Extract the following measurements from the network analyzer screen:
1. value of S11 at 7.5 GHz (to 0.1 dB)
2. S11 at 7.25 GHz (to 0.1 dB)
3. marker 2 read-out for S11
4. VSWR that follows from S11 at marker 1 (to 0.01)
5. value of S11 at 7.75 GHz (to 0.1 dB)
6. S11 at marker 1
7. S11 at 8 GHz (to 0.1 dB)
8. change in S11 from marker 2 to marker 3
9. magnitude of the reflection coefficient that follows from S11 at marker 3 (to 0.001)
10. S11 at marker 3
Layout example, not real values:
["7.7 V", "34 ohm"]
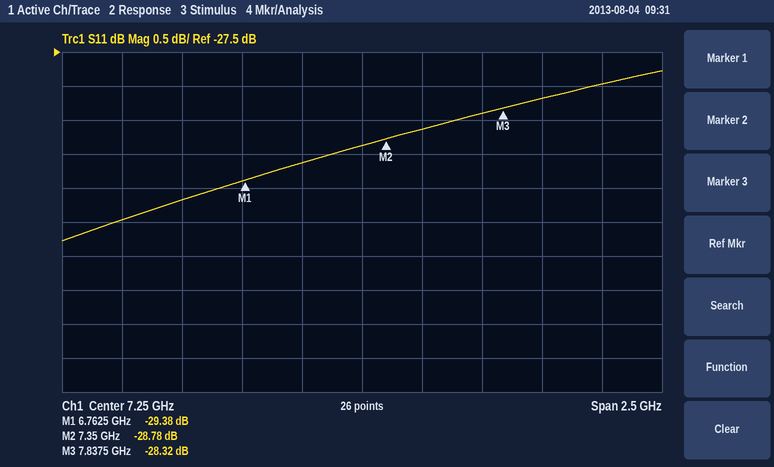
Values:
["-28.6 dB", "-28.9 dB", "-28.78 dB", "1.07", "-28.4 dB", "-29.38 dB", "-28.2 dB", "0.46 dB", "0.038", "-28.32 dB"]
